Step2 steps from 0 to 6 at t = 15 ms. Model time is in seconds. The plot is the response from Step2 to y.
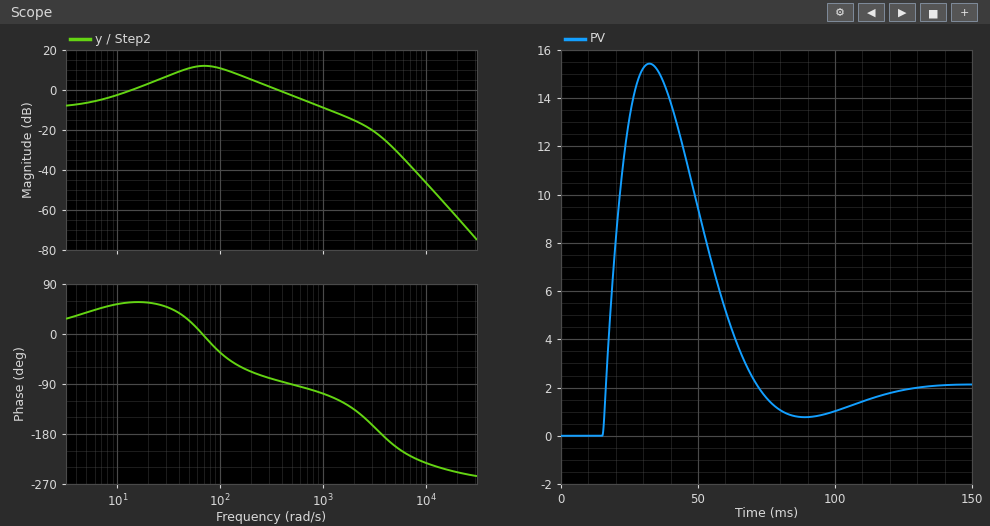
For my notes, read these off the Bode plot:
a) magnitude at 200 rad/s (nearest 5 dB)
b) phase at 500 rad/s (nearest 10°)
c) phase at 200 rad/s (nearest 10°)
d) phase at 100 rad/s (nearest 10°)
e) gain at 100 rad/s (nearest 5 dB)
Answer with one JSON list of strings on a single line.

["5 dB", "-90°", "-70°", "-30°", "10 dB"]
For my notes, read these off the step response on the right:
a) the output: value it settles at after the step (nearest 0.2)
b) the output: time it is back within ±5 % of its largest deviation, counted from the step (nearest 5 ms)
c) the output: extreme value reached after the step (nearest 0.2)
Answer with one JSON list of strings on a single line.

["2.2", "95 ms", "15.4"]
